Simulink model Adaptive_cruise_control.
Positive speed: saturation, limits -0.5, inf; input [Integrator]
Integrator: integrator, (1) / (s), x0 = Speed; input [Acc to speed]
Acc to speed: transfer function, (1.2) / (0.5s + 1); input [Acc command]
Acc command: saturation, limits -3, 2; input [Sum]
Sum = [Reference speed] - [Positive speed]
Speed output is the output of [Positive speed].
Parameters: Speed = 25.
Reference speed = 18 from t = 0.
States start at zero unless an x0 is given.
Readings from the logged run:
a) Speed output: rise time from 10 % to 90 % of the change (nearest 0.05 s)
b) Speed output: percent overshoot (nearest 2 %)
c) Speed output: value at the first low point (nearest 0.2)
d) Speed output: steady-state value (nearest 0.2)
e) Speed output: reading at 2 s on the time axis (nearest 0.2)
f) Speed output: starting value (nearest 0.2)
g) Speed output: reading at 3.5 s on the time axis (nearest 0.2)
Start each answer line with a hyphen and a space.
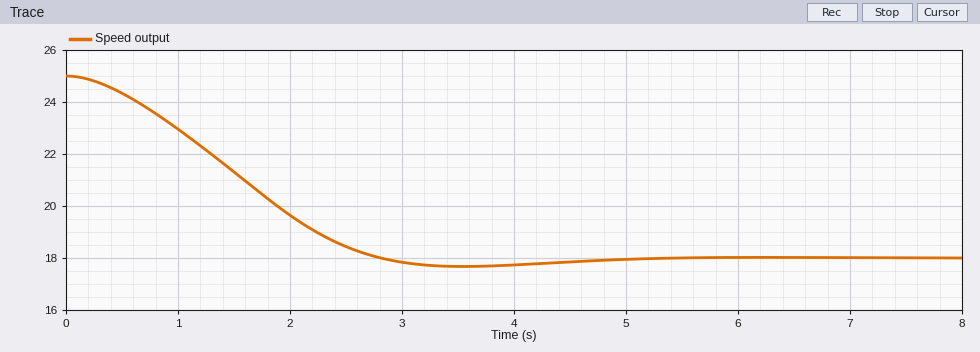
- 1.85 s
- 4 %
- 17.6
- 18.0
- 19.6
- 25.0
- 17.6
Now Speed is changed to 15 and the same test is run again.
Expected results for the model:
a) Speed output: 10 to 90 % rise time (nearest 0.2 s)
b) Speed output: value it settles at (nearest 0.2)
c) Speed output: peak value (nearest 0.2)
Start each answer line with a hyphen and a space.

- 1.4 s
- 18.0
- 18.2
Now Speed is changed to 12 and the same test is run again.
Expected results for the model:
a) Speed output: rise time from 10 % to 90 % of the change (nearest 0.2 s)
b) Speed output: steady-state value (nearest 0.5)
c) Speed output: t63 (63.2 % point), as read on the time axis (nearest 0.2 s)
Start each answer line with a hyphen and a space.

- 2.2 s
- 18.0
- 2.0 s
